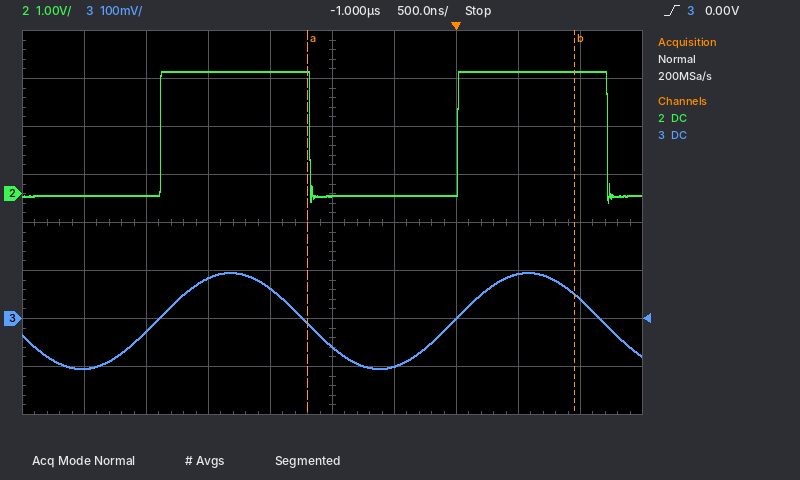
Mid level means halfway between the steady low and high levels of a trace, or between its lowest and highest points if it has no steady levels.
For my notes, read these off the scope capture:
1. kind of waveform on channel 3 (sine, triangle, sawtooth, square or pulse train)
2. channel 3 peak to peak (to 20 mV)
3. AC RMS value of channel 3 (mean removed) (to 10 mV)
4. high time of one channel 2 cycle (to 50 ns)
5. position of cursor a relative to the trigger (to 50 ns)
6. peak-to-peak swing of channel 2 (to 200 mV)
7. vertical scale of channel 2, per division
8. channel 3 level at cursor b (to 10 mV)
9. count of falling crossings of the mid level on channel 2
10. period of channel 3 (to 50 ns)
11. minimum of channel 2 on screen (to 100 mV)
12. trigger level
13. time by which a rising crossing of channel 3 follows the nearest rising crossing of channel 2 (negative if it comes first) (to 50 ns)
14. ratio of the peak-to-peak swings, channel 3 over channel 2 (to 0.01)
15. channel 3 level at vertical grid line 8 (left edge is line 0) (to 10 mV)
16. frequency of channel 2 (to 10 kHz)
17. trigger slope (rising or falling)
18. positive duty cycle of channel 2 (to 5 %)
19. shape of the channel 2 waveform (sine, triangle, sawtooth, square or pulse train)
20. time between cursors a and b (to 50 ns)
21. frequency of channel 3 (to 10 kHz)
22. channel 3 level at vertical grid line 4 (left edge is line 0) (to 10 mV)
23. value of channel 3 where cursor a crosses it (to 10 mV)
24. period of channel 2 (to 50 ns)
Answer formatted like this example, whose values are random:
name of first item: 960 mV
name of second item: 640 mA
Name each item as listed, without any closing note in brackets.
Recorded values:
kind of waveform on channel 3: sine
channel 3 peak to peak: 200 mV
AC RMS value of channel 3 (mean removed): 70 mV
high time of one channel 2 cycle: 1.20 µs
position of cursor a relative to the trigger: -1.20 µs
peak-to-peak swing of channel 2: 2.8 V
vertical scale of channel 2, per division: 1 V
channel 3 level at cursor b: 50 mV
count of falling crossings of the mid level on channel 2: 2
period of channel 3: 2.40 µs
minimum of channel 2 on screen: -200 mV
trigger level: 0.00 V
time by which a rising crossing of channel 3 follows the nearest rising crossing of channel 2 (negative if it comes first): -50 ns
ratio of the peak-to-peak swings, channel 3 over channel 2: 0.07
channel 3 level at vertical grid line 8 (left edge is line 0): 90 mV
frequency of channel 2: 420 kHz
trigger slope: rising
positive duty cycle of channel 2: 50 %
shape of the channel 2 waveform: square
time between cursors a and b: 2.15 µs
frequency of channel 3: 420 kHz
channel 3 level at vertical grid line 4 (left edge is line 0): 60 mV
value of channel 3 where cursor a crosses it: -10 mV
period of channel 2: 2.40 µs
